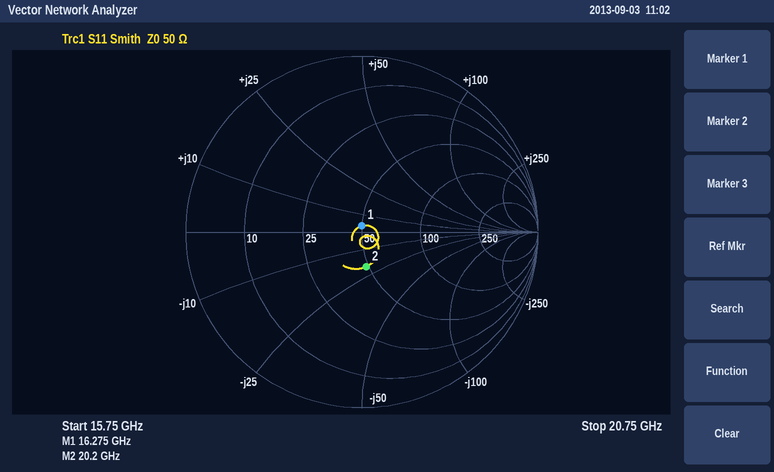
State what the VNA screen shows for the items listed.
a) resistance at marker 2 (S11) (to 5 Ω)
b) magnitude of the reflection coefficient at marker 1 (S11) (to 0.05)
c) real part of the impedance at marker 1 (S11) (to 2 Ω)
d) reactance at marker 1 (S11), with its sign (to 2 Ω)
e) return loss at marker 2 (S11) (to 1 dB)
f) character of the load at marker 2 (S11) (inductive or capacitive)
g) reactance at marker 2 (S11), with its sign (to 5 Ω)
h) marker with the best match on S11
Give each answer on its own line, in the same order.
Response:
50 Ω
0.05
50 Ω
+4 Ω
14 dB
capacitive
-20 Ω
marker 1
